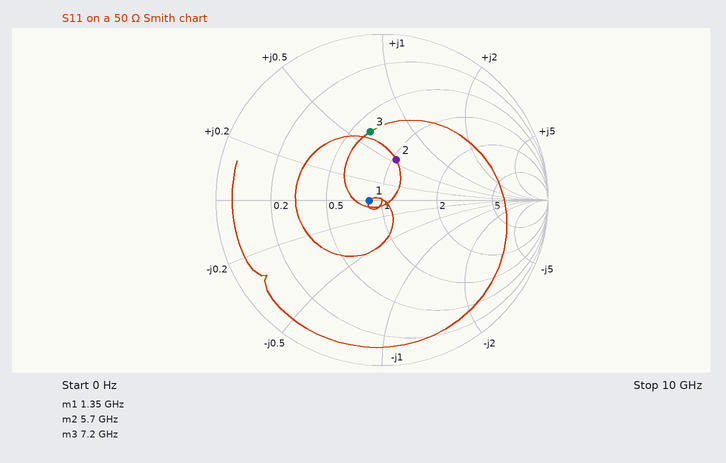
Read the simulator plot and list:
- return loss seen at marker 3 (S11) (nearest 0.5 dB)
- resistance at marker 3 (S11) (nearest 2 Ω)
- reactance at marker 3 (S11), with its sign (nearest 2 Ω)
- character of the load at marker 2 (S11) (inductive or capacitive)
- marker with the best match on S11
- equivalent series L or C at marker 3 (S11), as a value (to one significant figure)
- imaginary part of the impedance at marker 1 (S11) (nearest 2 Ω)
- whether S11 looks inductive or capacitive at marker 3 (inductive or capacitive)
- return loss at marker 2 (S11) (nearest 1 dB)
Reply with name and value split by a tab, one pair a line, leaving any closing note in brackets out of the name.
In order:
return loss seen at marker 3 (S11)	7.5 dB
resistance at marker 3 (S11)	32 Ω
reactance at marker 3 (S11), with its sign	+32 Ω
character of the load at marker 2 (S11)	inductive
marker with the best match on S11	marker 1
equivalent series L or C at marker 3 (S11), as a value	700 pH
imaginary part of the impedance at marker 1 (S11)	0 Ω
whether S11 looks inductive or capacitive at marker 3	inductive
return loss at marker 2 (S11)	12 dB
